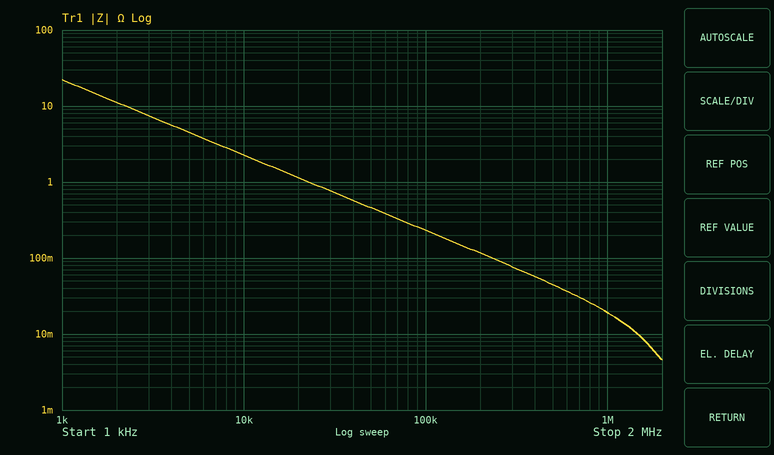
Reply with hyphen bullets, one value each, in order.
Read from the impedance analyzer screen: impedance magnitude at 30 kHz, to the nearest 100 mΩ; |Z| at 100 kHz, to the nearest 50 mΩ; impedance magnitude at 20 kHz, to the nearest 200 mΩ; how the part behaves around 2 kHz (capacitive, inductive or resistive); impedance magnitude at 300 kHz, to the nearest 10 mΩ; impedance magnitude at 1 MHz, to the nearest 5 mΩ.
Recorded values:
- 800 mΩ
- 250 mΩ
- 1.2 Ω
- capacitive
- 80 mΩ
- 20 mΩ
